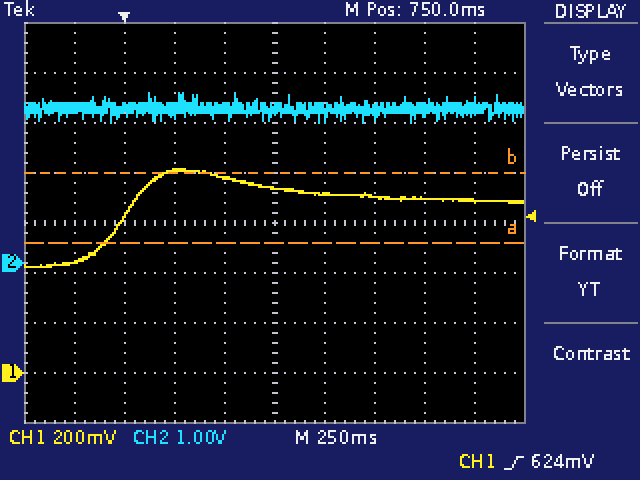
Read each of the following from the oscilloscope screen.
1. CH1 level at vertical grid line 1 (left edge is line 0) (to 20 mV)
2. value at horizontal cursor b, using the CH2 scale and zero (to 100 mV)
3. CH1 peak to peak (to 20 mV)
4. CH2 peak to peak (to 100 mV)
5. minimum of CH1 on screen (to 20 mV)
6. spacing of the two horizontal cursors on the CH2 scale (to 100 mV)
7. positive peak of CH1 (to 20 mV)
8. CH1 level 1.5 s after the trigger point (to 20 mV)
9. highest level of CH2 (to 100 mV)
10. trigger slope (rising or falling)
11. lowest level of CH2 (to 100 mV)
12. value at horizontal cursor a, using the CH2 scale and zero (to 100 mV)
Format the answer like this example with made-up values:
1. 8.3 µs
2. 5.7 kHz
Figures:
1. 440 mV
2. 1.8 V
3. 400 mV
4. 600 mV
5. 420 mV
6. 1.4 V
7. 820 mV
8. 700 mV
9. 3.4 V
10. rising
11. 2.8 V
12. 400 mV
